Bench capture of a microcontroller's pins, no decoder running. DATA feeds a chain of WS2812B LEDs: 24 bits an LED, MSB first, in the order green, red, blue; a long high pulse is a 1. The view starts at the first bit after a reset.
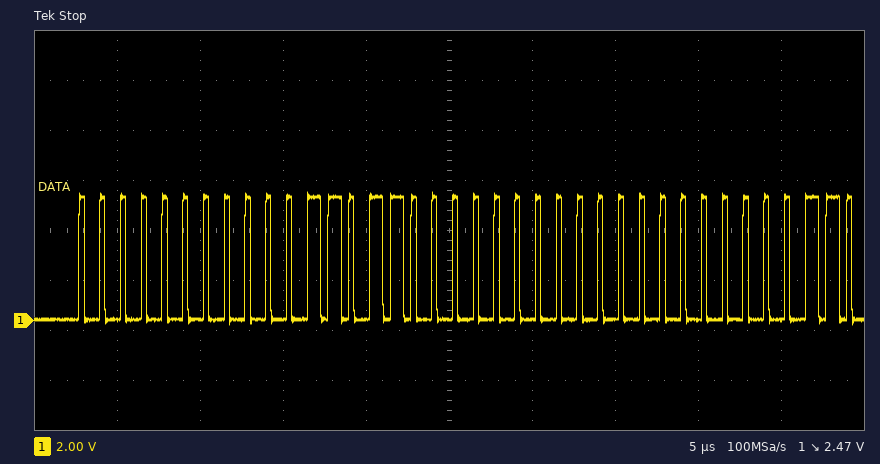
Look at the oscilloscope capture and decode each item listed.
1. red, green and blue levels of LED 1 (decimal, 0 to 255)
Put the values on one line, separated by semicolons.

27, 0, 0
